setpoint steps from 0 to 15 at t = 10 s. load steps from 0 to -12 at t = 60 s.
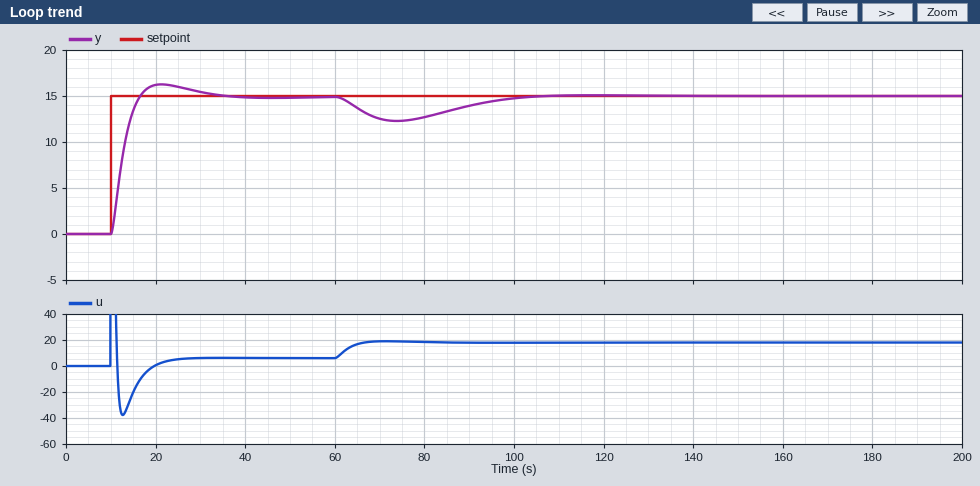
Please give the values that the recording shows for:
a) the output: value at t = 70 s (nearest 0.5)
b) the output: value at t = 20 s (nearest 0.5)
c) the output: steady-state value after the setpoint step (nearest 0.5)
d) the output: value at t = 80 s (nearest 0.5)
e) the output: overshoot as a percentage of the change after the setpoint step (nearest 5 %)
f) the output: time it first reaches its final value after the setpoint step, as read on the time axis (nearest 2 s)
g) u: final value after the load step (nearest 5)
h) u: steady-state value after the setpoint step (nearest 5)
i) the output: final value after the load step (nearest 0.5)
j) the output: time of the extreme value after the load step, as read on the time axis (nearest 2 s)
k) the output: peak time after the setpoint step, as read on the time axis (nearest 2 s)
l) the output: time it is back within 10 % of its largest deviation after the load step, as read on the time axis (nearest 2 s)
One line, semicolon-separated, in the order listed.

12.5; 16.0; 15.0; 12.5; 10 %; 16 s; 20; 5; 15.0; 74 s; 22 s; 100 s
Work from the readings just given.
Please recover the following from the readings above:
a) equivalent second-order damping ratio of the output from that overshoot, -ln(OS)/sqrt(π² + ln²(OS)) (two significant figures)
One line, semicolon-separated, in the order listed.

0.59
